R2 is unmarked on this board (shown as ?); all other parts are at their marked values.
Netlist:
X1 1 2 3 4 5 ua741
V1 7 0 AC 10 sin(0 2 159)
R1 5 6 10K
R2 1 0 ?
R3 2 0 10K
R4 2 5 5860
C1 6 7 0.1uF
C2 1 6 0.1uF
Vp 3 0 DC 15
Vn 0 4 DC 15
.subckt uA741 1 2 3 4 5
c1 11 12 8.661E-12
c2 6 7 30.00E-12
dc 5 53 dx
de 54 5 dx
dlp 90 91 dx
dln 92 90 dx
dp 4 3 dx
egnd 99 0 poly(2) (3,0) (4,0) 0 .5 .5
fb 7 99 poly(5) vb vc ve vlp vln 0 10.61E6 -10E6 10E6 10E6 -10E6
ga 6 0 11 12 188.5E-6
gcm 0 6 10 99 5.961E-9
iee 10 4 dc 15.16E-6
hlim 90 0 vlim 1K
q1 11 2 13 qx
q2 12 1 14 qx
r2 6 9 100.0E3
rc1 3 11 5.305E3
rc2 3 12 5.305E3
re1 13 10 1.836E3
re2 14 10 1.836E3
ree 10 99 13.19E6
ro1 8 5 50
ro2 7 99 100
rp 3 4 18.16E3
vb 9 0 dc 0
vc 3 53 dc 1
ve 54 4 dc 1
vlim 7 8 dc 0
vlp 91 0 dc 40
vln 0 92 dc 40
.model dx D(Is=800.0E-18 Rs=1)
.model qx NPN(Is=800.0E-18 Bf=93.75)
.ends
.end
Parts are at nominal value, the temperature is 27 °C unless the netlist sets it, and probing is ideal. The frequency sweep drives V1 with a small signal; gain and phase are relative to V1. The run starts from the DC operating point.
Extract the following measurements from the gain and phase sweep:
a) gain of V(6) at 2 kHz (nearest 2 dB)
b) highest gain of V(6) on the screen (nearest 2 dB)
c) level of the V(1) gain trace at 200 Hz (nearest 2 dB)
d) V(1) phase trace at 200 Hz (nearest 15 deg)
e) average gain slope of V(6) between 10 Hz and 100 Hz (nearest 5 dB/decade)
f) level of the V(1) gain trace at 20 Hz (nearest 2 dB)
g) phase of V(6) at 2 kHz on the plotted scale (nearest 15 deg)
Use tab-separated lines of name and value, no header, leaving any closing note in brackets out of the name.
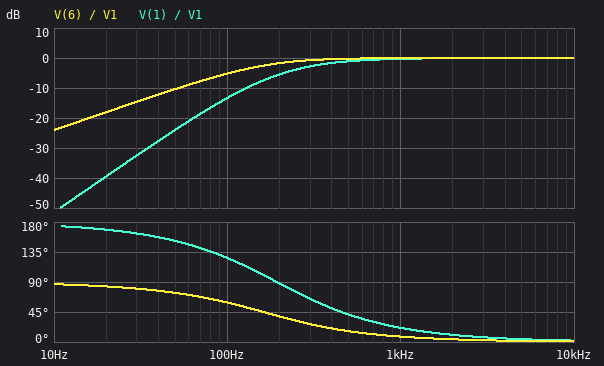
gain of V(6) at 2 kHz	0 dB
highest gain of V(6) on the screen	0 dB
level of the V(1) gain trace at 200 Hz	-6 dB
V(1) phase trace at 200 Hz	90 deg
average gain slope of V(6) between 10 Hz and 100 Hz	20 dB/decade
level of the V(1) gain trace at 20 Hz	-40 dB
phase of V(6) at 2 kHz on the plotted scale	0 deg
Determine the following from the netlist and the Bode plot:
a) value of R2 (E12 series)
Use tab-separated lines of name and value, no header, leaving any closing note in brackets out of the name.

value of R2	6.8 kΩ
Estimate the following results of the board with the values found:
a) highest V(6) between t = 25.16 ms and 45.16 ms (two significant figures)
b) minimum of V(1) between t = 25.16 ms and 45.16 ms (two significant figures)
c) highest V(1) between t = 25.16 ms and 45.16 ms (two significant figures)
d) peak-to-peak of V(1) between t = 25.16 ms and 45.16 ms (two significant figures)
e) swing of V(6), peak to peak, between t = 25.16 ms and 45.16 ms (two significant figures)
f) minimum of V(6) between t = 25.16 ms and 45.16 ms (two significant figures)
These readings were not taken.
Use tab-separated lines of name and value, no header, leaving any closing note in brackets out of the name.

highest V(6) between t = 25.16 ms and 45.16 ms	1.5 V
minimum of V(1) between t = 25.16 ms and 45.16 ms	-830 mV
highest V(1) between t = 25.16 ms and 45.16 ms	830 mV
peak-to-peak of V(1) between t = 25.16 ms and 45.16 ms	1.7 V
swing of V(6), peak to peak, between t = 25.16 ms and 45.16 ms	3.0 V
minimum of V(6) between t = 25.16 ms and 45.16 ms	-1.5 V
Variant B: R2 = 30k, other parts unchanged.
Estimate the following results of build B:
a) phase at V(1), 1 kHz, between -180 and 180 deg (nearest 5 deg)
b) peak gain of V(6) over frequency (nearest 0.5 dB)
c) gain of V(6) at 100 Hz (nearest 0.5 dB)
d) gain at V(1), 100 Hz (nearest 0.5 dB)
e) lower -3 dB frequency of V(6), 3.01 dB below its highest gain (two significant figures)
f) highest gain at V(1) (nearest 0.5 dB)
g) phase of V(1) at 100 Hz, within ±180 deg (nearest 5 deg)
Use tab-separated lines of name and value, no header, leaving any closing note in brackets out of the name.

phase at V(1), 1 kHz, between -180 and 180 deg	0 deg
peak gain of V(6) over frequency	18.5 dB
gain of V(6) at 100 Hz	15.0 dB
gain at V(1), 100 Hz	14.0 dB
lower -3 dB frequency of V(6), 3.01 dB below its highest gain	86 Hz
highest gain at V(1)	17.0 dB
phase of V(1) at 100 Hz, within ±180 deg	40 deg
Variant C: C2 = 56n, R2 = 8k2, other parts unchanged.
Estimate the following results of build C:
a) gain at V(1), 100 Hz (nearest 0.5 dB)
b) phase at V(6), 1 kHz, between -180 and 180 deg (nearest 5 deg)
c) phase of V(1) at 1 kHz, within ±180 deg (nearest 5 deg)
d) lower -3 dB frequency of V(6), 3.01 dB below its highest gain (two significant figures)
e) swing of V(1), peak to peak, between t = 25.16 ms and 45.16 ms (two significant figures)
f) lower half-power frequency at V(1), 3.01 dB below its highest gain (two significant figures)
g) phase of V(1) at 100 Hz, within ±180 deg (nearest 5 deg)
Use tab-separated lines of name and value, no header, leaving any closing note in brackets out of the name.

gain at V(1), 100 Hz	-16.0 dB
phase at V(6), 1 kHz, between -180 and 180 deg	5 deg
phase of V(1) at 1 kHz, within ±180 deg	25 deg
lower -3 dB frequency of V(6), 3.01 dB below its highest gain	140 Hz
swing of V(1), peak to peak, between t = 25.16 ms and 45.16 ms	1.3 V
lower half-power frequency at V(1), 3.01 dB below its highest gain	340 Hz
phase of V(1) at 100 Hz, within ±180 deg	135 deg
